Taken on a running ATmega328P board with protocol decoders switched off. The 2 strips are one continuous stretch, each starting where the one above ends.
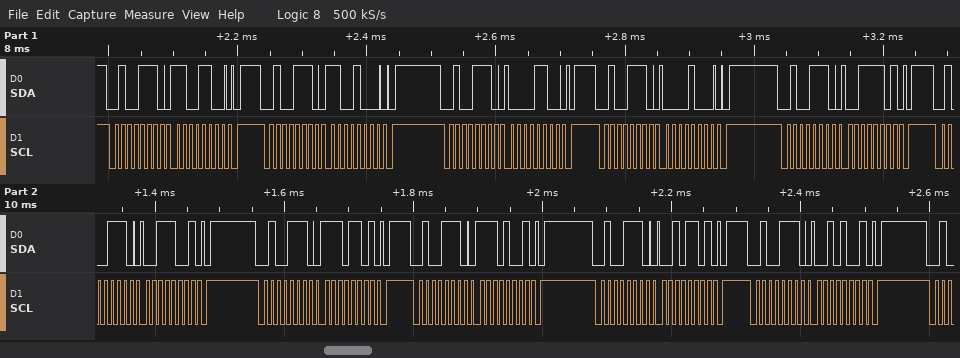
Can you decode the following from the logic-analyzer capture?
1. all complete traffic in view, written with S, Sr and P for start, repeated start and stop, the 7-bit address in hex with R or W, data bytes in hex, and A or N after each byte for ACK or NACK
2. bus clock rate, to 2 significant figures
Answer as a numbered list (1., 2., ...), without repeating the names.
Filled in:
1. S 27W A CC A P S 27W A C8 A P S 27W A 0C A P S 27W A 08 A P S 27W A 3D A P S 27W A 39 A P S 27W A ED A P S 27W A E9 A P S 27W A 2D A P S 27W A 29 A P
2. 100 kHz
